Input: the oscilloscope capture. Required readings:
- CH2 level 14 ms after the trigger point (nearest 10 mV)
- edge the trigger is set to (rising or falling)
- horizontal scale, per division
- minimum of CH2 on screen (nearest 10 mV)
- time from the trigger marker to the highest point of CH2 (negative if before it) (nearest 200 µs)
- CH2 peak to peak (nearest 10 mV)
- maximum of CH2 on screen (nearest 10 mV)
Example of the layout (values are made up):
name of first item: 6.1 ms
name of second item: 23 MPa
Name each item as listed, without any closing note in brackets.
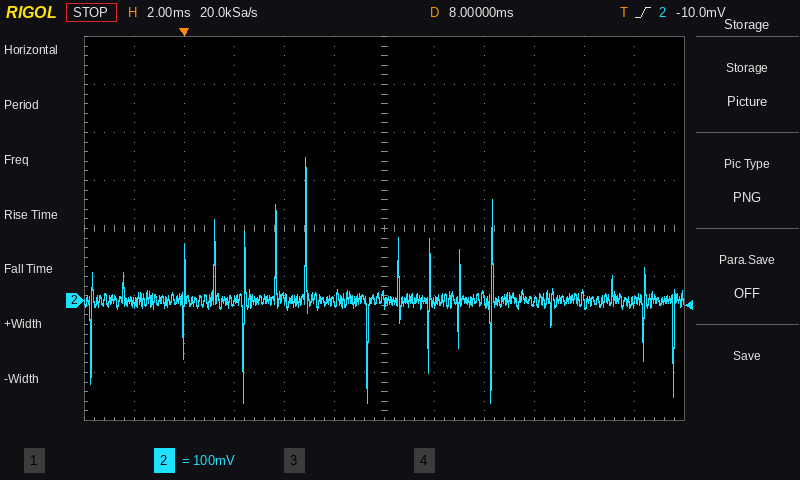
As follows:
CH2 level 14 ms after the trigger point: 0 mV
edge the trigger is set to: rising
horizontal scale, per division: 2 ms
minimum of CH2 on screen: -210 mV
time from the trigger marker to the highest point of CH2 (negative if before it): +4.8 ms
CH2 peak to peak: 510 mV
maximum of CH2 on screen: 300 mV
